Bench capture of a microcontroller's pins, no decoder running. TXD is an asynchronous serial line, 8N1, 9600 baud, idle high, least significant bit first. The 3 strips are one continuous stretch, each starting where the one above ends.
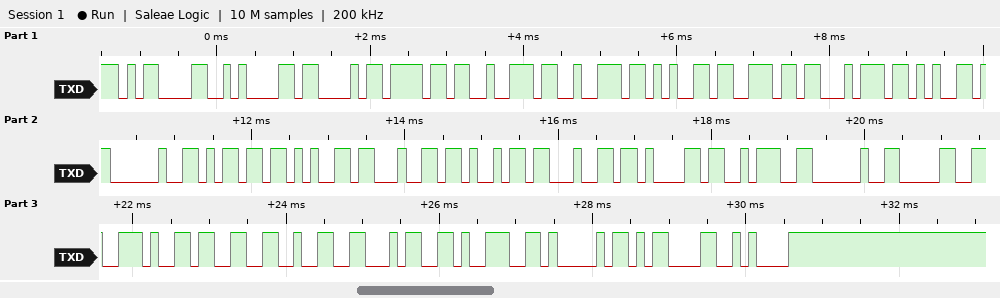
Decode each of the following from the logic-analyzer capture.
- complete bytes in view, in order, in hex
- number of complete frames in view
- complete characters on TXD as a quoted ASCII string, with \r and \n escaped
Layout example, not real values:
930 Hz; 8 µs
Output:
0D 0A 43 6F 72 72 65 6E 74 65 20 6D 65 64 69 64 61 3A 20 30 2E 33 32 34 39 41 0D 0A; 28; "\r\nCorrente medida: 0.3249A\r\n"
